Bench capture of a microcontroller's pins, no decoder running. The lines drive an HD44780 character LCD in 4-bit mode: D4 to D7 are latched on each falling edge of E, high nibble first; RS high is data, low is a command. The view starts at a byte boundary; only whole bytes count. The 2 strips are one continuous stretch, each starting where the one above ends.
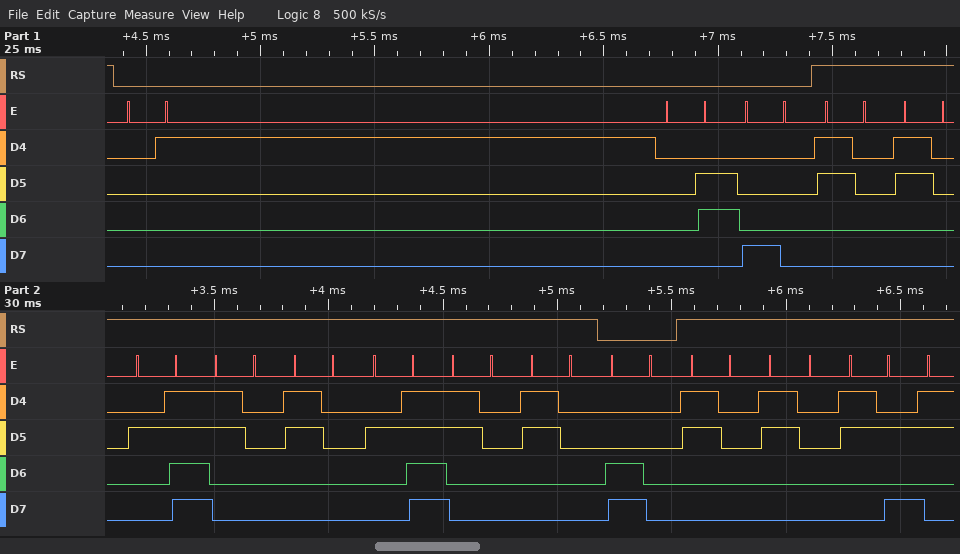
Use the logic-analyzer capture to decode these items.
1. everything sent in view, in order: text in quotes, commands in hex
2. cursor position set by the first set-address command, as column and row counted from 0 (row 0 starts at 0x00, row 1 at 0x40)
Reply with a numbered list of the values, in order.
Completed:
1. 0x01 0x06 0x80 "00/00/00" 0xC0 "00:"
2. column 0, row 0
